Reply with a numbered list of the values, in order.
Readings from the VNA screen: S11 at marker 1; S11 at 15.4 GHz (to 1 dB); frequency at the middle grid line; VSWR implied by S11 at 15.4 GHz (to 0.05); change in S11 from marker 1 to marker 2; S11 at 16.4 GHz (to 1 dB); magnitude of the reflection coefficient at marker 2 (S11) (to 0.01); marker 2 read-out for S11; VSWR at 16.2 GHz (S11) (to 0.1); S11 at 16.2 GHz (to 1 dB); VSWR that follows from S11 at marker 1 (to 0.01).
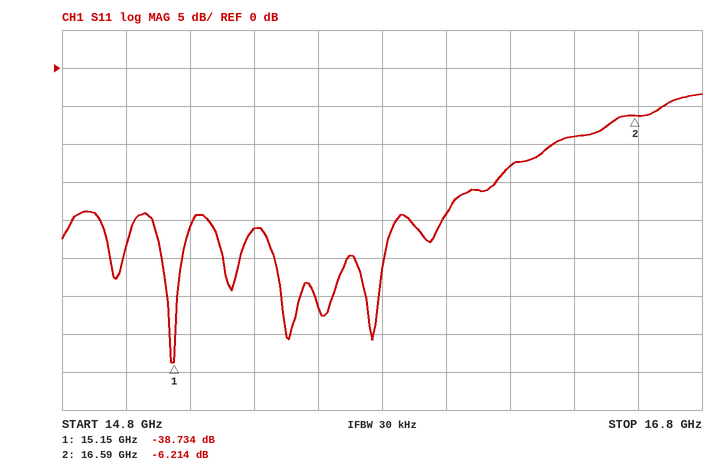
1. -38.734 dB
2. -21 dB
3. 15.8 GHz
4. 1.20
5. 32.520 dB
6. -9 dB
7. 0.49
8. -6.214 dB
9. 1.6
10. -13 dB
11. 1.02
